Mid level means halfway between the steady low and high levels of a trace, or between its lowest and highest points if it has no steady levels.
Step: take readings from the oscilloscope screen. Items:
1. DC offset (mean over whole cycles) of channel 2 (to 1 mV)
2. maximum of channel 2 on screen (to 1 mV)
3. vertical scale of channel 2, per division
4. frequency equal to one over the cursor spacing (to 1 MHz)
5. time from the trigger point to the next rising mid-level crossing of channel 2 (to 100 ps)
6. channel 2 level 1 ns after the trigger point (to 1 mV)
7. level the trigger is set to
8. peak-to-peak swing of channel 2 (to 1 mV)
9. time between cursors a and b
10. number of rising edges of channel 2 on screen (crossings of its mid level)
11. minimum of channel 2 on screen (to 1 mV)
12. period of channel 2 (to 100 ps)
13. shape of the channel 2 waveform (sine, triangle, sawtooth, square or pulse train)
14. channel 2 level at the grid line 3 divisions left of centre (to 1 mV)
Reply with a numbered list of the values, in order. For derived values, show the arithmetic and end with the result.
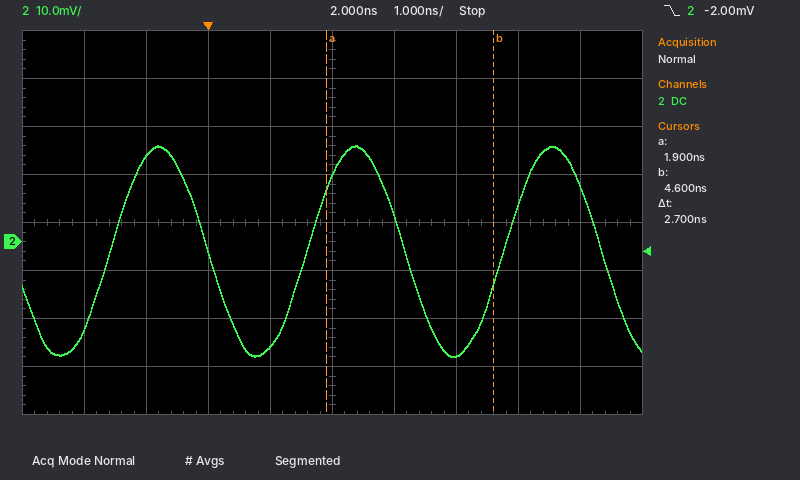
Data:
1. (20 mV + (-24 mV)) / 2 ≈ -2 mV
2. 20 mV
3. 10 mV
4. 1 / 2.7 ns ≈ 370 MHz
5. 1.6 ns
6. -22 mV
7. -2.00 mV
8. 20 mV − (-24 mV) = 44 mV
9. 2.7 ns
10. 3
11. -24 mV
12. 3.2 ns
13. sine
14. 18 mV
